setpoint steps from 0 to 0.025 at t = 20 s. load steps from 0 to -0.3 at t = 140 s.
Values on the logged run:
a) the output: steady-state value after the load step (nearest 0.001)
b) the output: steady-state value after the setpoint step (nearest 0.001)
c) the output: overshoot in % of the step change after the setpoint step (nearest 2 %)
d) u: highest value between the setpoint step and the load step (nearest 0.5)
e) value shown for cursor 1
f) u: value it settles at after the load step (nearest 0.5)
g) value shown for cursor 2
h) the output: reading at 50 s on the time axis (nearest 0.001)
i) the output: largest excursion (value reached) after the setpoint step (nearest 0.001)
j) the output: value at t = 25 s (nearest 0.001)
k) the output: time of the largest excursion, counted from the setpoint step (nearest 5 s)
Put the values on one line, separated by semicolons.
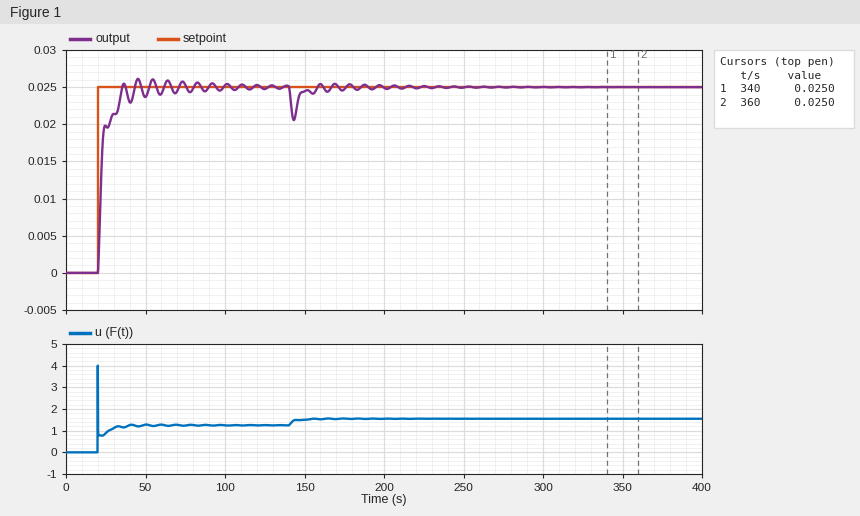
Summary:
0.025; 0.025; 4 %; 4.0; 0.0250; 1.5; 0.0250; 0.024; 0.026; 0.020; 25 s
